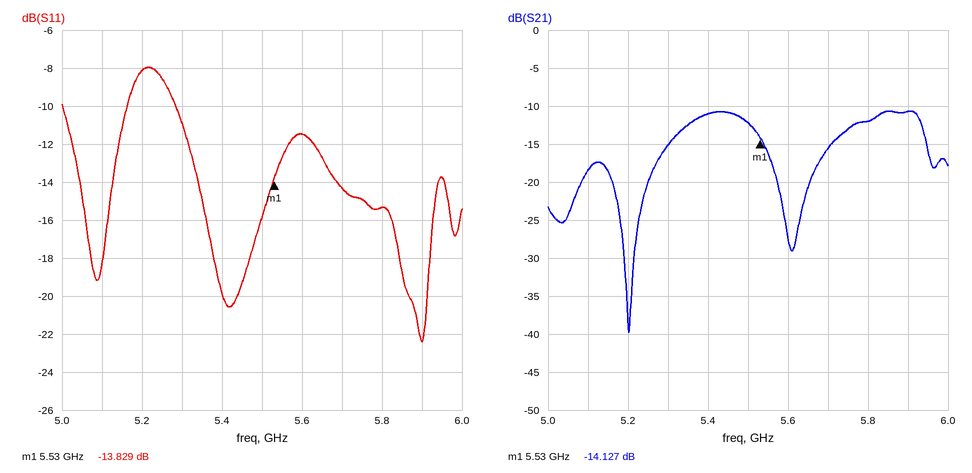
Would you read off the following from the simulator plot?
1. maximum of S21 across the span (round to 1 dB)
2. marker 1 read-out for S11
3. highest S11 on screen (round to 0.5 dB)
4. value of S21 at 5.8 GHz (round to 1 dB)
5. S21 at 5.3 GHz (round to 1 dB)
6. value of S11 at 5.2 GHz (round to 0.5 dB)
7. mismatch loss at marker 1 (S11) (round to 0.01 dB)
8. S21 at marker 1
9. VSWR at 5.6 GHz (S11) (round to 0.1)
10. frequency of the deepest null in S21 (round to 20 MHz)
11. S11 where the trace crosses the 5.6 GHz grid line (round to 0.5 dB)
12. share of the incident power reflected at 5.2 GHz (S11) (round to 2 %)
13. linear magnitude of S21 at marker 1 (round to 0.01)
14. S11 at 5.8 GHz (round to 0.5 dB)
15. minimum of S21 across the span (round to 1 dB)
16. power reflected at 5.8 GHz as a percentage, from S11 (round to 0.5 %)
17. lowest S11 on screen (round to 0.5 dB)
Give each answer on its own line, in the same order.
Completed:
-11 dB
-13.829 dB
-8.0 dB
-12 dB
-15 dB
-8.0 dB
0.18 dB
-14.127 dB
1.7
5.20 GHz
-11.5 dB
16 %
0.20
-15.5 dB
-40 dB
3.0 %
-22.5 dB
